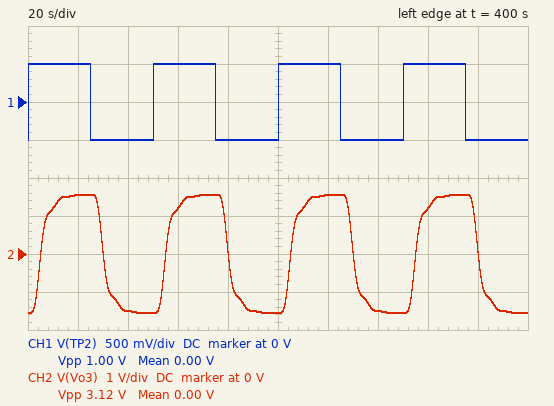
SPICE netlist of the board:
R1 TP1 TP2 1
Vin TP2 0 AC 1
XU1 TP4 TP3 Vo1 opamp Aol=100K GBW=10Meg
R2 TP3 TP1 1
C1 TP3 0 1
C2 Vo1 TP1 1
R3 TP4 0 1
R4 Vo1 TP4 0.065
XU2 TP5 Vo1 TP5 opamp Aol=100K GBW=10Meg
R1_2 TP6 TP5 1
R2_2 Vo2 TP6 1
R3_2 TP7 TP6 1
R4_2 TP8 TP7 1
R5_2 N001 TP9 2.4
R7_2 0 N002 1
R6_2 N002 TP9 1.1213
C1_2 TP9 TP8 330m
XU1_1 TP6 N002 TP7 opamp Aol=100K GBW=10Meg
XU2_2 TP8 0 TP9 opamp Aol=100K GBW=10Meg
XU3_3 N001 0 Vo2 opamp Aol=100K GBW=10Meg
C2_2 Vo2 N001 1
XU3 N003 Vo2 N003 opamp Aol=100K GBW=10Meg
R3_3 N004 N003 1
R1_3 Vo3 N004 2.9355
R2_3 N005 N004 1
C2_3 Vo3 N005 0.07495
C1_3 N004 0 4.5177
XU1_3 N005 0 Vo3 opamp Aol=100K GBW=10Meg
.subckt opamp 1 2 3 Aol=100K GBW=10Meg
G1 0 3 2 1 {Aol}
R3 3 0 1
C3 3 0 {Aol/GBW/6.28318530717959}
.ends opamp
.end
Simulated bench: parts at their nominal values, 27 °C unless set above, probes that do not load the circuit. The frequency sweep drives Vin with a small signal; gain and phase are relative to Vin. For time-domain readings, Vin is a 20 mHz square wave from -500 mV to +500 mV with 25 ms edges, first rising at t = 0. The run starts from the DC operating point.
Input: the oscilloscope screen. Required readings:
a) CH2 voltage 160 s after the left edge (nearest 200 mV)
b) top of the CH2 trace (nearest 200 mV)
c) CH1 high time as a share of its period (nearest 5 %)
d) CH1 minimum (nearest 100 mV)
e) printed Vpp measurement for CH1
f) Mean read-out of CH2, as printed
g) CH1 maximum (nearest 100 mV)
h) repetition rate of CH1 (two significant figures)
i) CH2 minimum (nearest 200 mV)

1.2 V
1.6 V
50 %
-500 mV
1.00 V
0.00 V
500 mV
20 mHz
-1.6 V
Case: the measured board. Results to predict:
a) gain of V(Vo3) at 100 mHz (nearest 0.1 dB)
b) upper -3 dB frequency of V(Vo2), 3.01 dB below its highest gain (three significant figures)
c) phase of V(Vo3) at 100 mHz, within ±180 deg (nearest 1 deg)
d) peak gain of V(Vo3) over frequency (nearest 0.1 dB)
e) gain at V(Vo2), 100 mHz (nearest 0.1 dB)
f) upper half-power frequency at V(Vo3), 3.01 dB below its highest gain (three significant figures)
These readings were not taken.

3.5 dB
43.8 mHz
-164 deg
9.9 dB
-9.1 dB
50.7 mHz
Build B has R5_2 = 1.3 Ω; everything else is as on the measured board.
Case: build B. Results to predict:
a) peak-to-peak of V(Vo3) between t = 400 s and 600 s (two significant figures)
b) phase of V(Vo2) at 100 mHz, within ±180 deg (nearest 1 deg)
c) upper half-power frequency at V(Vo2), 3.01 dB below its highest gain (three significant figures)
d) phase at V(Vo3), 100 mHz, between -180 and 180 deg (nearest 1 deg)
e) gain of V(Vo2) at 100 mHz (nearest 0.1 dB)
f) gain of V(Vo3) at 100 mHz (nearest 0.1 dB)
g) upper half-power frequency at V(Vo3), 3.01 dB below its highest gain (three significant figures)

3.2 V
62 deg
68.5 mHz
-146 deg
-5.2 dB
7.4 dB
123 mHz
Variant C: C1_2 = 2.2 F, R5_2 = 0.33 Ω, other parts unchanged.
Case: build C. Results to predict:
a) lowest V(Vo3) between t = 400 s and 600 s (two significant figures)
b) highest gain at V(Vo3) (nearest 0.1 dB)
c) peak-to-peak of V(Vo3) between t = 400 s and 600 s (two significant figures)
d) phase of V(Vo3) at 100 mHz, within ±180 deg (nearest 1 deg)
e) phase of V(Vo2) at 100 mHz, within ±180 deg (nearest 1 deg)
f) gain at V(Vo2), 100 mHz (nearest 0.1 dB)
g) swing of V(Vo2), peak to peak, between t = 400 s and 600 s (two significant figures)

-2.8 V
15.7 dB
5.7 V
-114 deg
94 deg
0.1 dB
1.3 V
